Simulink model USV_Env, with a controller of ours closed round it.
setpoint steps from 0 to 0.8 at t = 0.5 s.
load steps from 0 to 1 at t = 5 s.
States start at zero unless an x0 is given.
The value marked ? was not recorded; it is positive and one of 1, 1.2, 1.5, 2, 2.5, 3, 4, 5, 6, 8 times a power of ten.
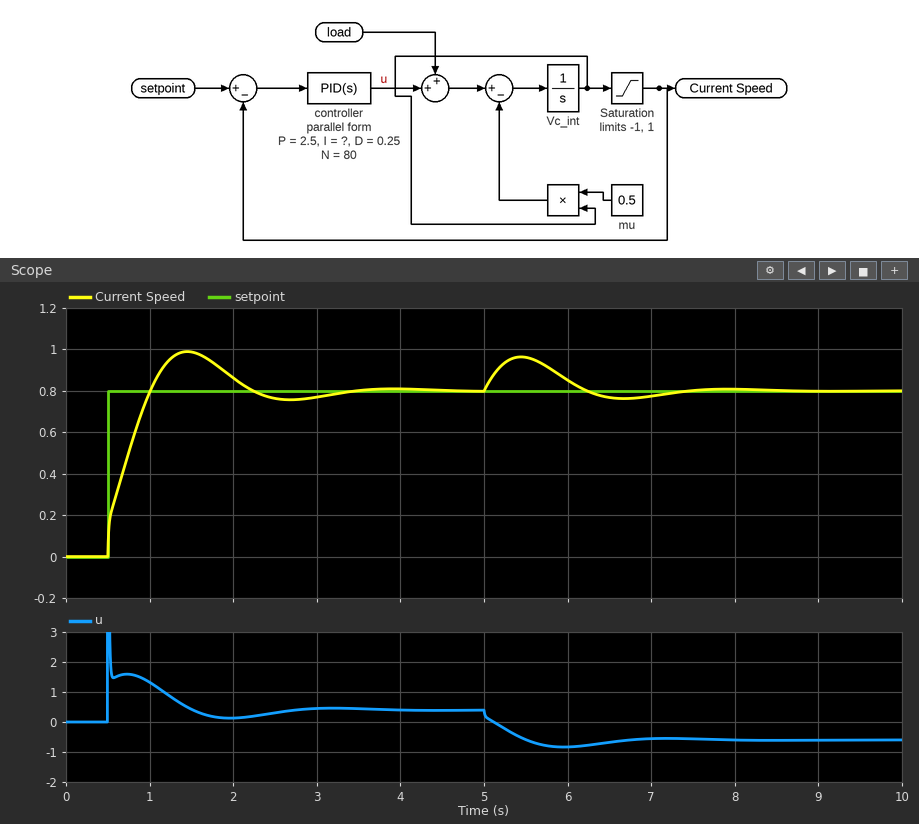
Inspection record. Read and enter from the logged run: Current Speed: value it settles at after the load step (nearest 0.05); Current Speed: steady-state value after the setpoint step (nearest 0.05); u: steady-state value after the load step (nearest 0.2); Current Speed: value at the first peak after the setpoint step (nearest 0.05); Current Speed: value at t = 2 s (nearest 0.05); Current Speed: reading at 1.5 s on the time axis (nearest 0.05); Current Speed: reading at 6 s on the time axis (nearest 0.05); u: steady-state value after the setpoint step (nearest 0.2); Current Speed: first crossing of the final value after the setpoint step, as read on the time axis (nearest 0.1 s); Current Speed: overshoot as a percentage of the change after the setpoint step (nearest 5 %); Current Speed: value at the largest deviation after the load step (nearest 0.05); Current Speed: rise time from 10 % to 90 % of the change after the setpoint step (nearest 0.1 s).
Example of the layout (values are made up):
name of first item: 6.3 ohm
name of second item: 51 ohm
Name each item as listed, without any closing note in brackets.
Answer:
Current Speed: value it settles at after the load step: 0.80
Current Speed: steady-state value after the setpoint step: 0.80
u: steady-state value after the load step: -0.6
Current Speed: value at the first peak after the setpoint step: 1.00
Current Speed: value at t = 2 s: 0.85
Current Speed: reading at 1.5 s on the time axis: 1.00
Current Speed: reading at 6 s on the time axis: 0.85
u: steady-state value after the setpoint step: 0.4
Current Speed: first crossing of the final value after the setpoint step, as read on the time axis: 1.0 s
Current Speed: overshoot as a percentage of the change after the setpoint step: 25 %
Current Speed: value at the largest deviation after the load step: 0.95
Current Speed: rise time from 10 % to 90 % of the change after the setpoint step: 0.4 s
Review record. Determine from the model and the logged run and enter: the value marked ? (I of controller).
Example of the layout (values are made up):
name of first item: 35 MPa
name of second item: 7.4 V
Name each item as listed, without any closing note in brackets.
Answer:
the value marked ?: 10
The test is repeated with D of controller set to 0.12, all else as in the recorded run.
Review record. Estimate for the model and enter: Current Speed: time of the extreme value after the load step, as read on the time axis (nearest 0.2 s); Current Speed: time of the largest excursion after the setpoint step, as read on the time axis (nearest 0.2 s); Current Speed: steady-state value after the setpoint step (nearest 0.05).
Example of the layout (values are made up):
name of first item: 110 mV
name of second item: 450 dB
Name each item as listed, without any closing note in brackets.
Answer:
Current Speed: time of the extreme value after the load step, as read on the time axis: 5.4 s
Current Speed: time of the largest excursion after the setpoint step, as read on the time axis: 1.4 s
Current Speed: steady-state value after the setpoint step: 0.80
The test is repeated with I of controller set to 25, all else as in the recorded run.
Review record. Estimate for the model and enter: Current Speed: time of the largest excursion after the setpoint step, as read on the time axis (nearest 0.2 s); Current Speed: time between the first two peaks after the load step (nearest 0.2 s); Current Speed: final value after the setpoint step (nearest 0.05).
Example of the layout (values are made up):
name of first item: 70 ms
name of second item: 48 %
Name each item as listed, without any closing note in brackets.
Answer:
Current Speed: time of the largest excursion after the setpoint step, as read on the time axis: 1.0 s
Current Speed: time between the first two peaks after the load step: 1.4 s
Current Speed: final value after the setpoint step: 0.80
